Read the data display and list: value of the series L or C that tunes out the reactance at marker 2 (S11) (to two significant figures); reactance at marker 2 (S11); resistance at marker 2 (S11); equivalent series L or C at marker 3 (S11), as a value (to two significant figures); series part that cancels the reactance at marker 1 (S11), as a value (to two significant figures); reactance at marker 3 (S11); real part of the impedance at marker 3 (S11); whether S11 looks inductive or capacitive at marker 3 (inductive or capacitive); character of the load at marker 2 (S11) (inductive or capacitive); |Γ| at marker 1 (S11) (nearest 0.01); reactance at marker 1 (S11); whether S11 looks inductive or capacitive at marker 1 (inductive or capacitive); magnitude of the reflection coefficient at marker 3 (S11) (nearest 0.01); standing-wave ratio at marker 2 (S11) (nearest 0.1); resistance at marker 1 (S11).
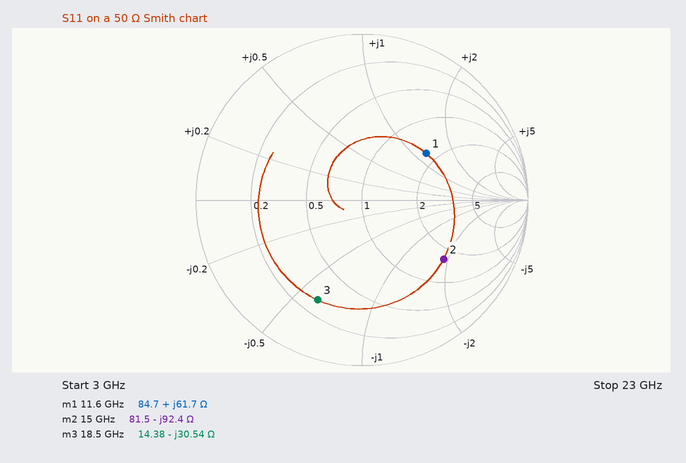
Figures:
980 pH
-92.4 Ω
81.5 Ω
280 fF
220 fF
-30.54 Ω
14.38 Ω
capacitive
capacitive
0.48
+61.7 Ω
inductive
0.66
4.1
84.7 Ω
